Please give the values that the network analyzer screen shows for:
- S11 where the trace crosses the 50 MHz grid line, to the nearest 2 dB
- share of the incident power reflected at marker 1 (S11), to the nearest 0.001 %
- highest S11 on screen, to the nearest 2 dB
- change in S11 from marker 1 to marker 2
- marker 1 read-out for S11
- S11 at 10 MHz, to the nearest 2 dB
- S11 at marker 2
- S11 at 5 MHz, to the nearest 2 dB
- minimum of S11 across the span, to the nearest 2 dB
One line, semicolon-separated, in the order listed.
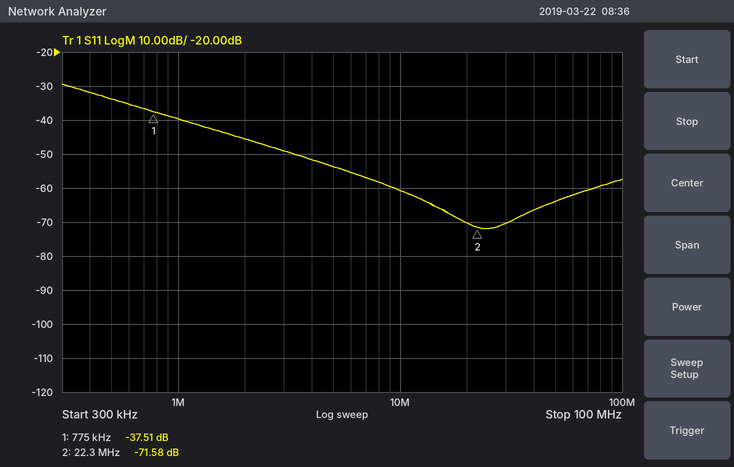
-64 dB; 0.018 %; -30 dB; -34.07 dB; -37.51 dB; -60 dB; -71.58 dB; -54 dB; -72 dB
